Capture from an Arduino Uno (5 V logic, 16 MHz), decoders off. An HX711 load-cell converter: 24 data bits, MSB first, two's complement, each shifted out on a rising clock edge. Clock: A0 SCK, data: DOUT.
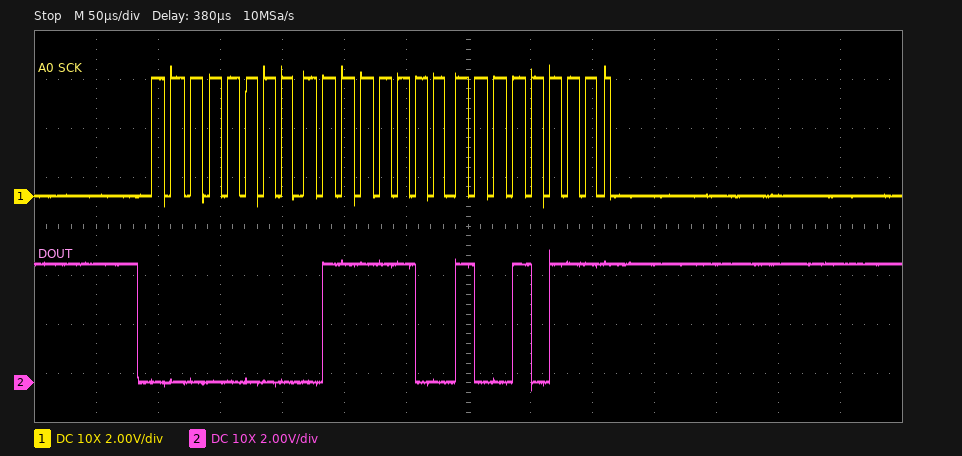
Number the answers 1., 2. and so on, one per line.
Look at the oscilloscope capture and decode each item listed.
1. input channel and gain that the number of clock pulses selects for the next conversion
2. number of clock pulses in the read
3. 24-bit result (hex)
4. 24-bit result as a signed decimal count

1. channel A, gain 128
2. 25
3. 0x007C97
4. 31895
